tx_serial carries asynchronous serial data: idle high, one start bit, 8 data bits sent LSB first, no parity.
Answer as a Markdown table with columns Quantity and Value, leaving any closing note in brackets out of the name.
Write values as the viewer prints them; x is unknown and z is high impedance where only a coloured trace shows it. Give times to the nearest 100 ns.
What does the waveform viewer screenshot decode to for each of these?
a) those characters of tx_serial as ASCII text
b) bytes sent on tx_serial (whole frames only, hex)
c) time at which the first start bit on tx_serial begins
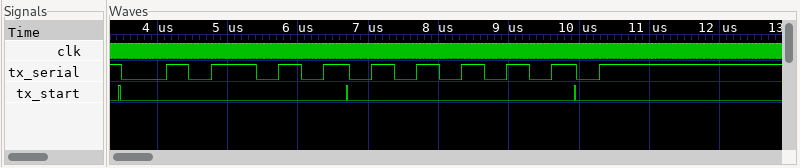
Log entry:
| Quantity | Value |
|---|---|
| those characters of tx_serial as ASCII text | "ZU" |
| bytes sent on tx_serial | 5A, 55 |
| time at which the first start bit on tx_serial begins | 3500 ns |
